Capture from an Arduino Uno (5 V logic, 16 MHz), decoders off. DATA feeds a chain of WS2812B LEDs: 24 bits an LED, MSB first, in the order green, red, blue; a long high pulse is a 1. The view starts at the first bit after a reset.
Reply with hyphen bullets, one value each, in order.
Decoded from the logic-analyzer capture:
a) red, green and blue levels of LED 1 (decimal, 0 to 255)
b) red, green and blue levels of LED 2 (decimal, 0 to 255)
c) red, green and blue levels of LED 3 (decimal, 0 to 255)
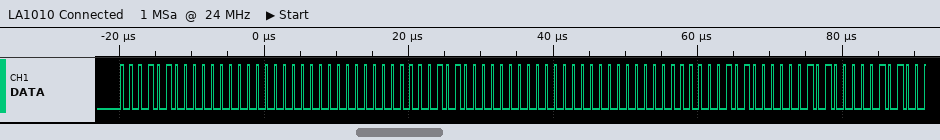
- 0, 20, 0
- 20, 0, 0
- 0, 0, 20
